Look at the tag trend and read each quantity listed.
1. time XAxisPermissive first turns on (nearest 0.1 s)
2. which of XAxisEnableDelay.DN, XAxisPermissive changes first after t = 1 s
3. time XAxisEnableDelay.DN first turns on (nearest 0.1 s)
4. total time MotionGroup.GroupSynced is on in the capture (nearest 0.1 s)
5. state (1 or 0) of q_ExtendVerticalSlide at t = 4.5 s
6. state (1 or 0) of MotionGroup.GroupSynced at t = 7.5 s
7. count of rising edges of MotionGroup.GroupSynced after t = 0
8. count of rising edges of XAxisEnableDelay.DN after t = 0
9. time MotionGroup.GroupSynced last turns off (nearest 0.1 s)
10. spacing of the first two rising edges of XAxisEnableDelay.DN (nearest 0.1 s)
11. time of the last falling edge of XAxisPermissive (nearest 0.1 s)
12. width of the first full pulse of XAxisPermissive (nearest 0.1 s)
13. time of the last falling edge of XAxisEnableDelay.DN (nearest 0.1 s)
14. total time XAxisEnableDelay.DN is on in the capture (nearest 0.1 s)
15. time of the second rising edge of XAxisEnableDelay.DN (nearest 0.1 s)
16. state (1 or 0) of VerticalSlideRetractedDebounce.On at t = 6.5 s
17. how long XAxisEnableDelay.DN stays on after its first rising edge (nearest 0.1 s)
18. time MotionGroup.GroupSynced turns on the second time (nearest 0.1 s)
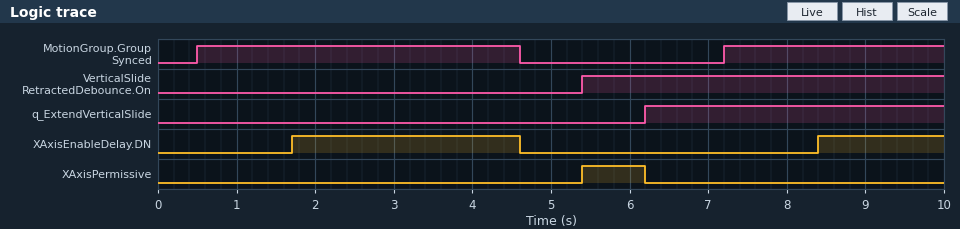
5.4 s
XAxisEnableDelay.DN
1.7 s
6.9 s
0
1
2
2
4.6 s
6.7 s
6.2 s
0.8 s
4.6 s
4.5 s
8.4 s
1
2.9 s
7.2 s
